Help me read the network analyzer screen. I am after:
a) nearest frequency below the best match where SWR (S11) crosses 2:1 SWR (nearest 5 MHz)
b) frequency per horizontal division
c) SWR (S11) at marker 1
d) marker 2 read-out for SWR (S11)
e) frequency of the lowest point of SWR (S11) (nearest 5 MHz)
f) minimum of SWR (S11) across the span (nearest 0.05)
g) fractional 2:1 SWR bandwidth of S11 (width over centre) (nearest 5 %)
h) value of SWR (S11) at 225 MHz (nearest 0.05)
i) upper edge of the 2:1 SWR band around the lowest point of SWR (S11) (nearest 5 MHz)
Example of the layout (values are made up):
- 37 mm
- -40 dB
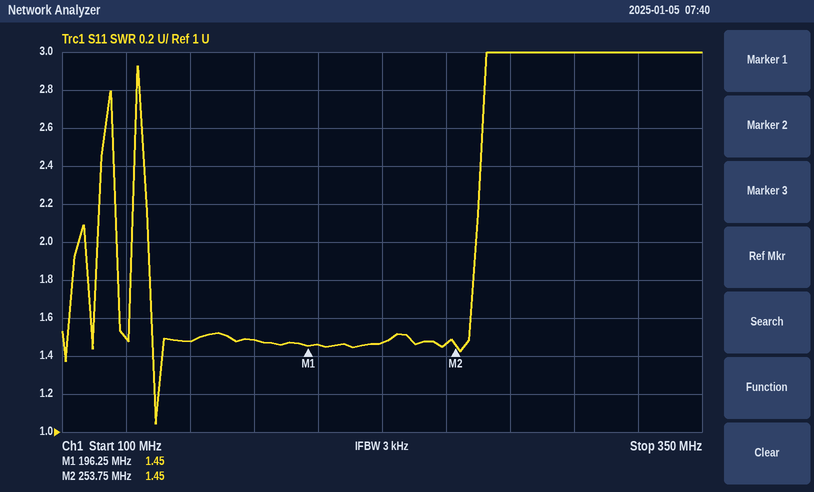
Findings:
- 135 MHz
- 25 MHz
- 1.45
- 1.45
- 135 MHz
- 1.05
- 65 %
- 1.45
- 260 MHz
